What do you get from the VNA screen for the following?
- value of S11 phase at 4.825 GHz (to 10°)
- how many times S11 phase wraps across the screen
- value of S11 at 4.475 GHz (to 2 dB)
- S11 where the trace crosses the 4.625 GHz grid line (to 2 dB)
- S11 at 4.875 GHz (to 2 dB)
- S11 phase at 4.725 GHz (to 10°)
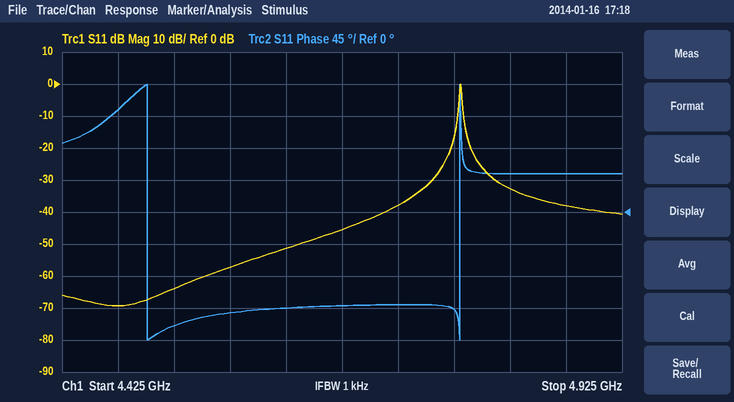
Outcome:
50°
2
-70 dB
-52 dB
-38 dB
-130°
